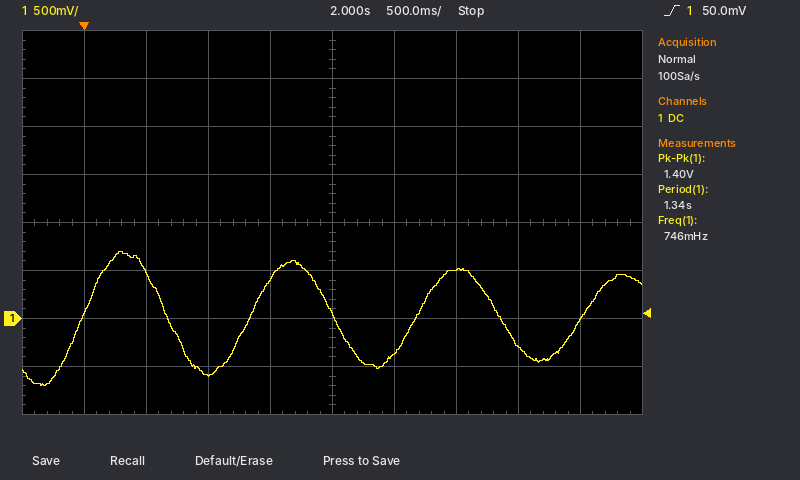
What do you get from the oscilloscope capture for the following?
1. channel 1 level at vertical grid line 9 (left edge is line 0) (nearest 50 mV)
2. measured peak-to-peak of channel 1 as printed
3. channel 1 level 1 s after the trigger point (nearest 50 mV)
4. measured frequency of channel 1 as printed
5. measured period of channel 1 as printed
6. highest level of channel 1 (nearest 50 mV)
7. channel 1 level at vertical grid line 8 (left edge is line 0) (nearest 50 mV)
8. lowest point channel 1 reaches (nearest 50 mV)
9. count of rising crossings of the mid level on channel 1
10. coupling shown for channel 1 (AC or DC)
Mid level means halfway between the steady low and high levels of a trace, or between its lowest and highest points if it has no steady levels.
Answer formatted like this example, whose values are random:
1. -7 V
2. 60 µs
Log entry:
1. 0 mV
2. 1.40 V
3. -600 mV
4. 746 mHz
5. 1.34 s
6. 700 mV
7. -300 mV
8. -700 mV
9. 4
10. DC
